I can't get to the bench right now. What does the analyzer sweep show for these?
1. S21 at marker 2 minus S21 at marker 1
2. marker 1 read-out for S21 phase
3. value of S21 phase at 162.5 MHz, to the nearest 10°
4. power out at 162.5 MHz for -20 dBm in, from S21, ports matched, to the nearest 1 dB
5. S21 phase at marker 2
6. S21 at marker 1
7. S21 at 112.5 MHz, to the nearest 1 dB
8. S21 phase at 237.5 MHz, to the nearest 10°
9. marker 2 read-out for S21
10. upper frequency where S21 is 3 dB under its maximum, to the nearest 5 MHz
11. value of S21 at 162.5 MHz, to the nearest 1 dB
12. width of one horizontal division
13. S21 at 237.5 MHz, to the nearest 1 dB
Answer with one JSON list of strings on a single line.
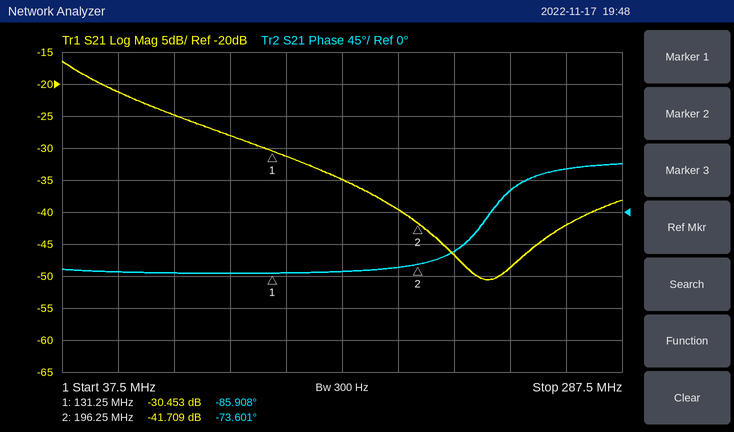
["-11.256 dB", "-85.908°", "-80°", "-55 dBm", "-73.601°", "-30.453 dB", "-28 dB", "30°", "-41.709 dB", "50 MHz", "-35 dB", "25 MHz", "-49 dB"]
